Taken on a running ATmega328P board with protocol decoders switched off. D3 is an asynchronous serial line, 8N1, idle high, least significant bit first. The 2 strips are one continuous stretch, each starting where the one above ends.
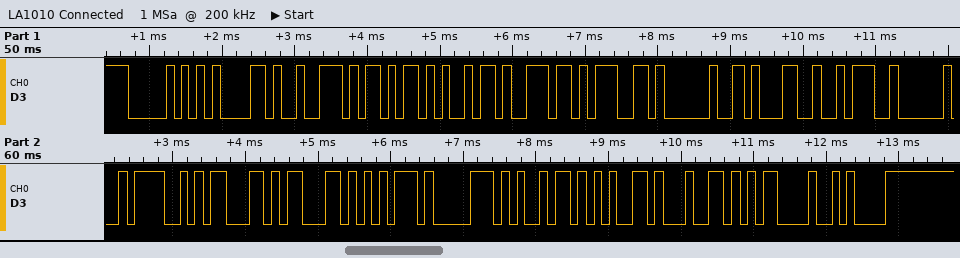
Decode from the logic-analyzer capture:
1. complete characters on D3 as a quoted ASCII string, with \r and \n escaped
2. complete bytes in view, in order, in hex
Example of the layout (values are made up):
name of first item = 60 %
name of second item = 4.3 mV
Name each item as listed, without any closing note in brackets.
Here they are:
complete characters on D3 as a quoted ASCII string, with \r and \n escaped = "Parking 1: Occupied\r\n"
complete bytes in view, in order, in hex = 50 61 72 6B 69 6E 67 20 31 3A 20 4F 63 63 75 70 69 65 64 0D 0A
